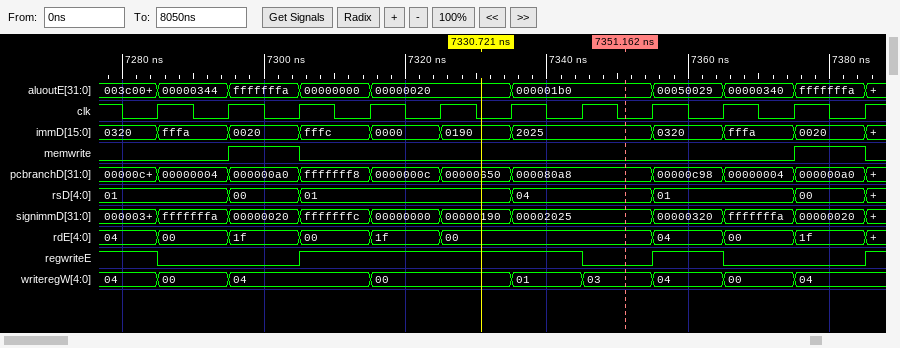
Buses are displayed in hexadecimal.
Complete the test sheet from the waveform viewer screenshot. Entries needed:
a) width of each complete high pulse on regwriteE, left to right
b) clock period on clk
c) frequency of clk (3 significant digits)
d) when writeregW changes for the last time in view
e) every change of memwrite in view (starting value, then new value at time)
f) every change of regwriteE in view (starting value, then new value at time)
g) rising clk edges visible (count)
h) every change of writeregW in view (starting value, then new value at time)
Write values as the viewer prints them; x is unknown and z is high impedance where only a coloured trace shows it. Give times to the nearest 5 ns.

40 ns, 10 ns
10 ns
100 MHz
7375 ns
0, 1 at 7295 ns, 0 at 7305 ns, 1 at 7375 ns, 0 at 7385 ns
1, 0 at 7285 ns, 1 at 7305 ns, 0 at 7345 ns, 1 at 7355 ns, 0 at 7365 ns, 1 at 7385 ns
11
04, 00 at 7285 ns, 04 at 7295 ns, 00 at 7315 ns, 01 at 7335 ns, 03 at 7345 ns, 04 at 7355 ns, 00 at 7365 ns, 04 at 7375 ns
